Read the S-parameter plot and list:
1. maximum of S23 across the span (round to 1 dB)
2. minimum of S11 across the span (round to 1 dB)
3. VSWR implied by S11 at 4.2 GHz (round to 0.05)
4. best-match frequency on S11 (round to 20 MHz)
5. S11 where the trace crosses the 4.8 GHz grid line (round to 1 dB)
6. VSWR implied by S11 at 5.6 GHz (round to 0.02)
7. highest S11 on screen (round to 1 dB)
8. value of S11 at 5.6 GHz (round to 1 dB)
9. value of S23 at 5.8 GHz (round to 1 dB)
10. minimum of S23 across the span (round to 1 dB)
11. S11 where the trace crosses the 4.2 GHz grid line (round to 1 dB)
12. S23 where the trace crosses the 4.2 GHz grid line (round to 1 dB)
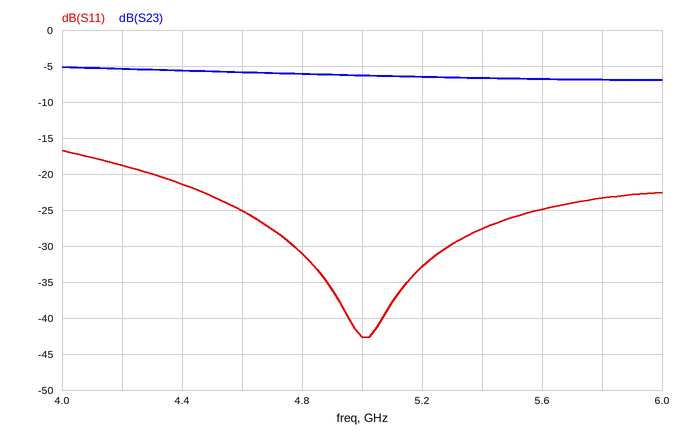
-5 dB
-43 dB
1.25
5.00 GHz
-31 dB
1.12
-17 dB
-25 dB
-7 dB
-7 dB
-19 dB
-5 dB
